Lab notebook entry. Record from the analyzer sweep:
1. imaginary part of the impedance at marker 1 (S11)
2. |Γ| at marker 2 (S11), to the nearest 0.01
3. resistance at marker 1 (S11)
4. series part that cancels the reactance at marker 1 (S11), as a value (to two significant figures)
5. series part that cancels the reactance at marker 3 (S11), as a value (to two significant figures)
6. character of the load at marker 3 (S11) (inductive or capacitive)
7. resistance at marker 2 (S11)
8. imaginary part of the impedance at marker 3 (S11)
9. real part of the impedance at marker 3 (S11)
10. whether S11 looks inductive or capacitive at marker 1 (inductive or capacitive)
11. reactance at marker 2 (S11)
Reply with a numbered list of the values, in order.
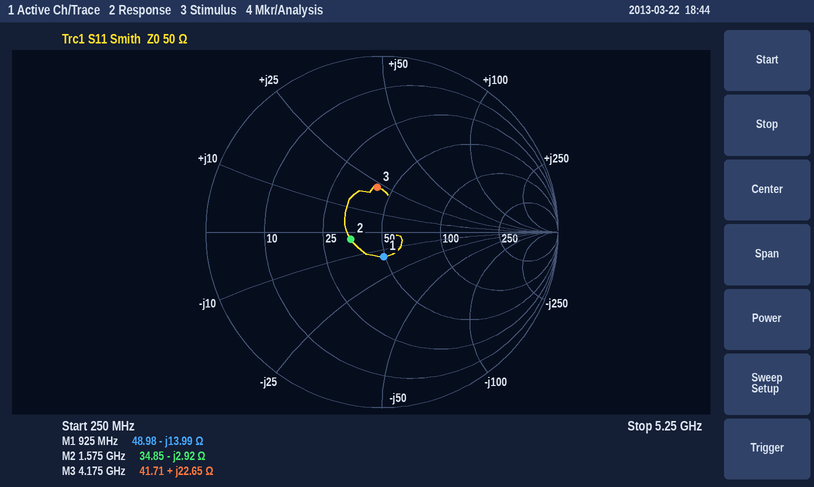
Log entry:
1. -13.99 Ω
2. 0.18
3. 48.98 Ω
4. 2.4 nH
5. 1.7 pF
6. inductive
7. 34.85 Ω
8. +22.65 Ω
9. 41.71 Ω
10. capacitive
11. -2.92 Ω
